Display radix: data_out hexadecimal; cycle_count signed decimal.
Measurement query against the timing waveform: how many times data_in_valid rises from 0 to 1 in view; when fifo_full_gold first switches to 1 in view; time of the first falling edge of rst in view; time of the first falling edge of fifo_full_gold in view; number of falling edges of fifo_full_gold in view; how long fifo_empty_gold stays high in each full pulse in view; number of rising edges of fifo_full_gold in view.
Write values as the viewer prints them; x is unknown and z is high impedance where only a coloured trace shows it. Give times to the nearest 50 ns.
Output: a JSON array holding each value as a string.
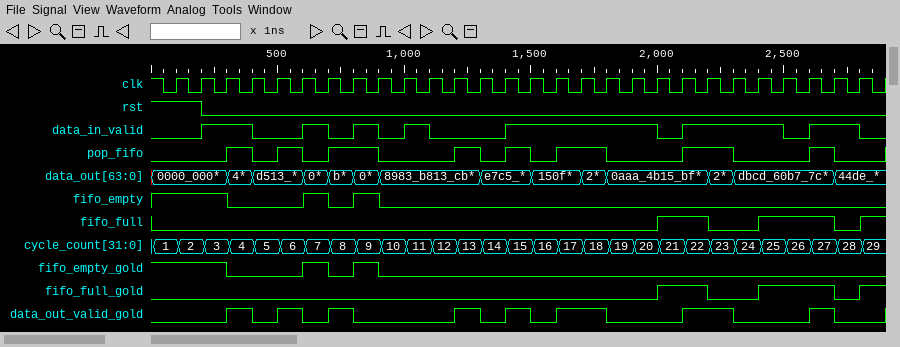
["7", "2000 ns", "200 ns", "2200 ns", "2", "100 ns, 100 ns", "3"]
